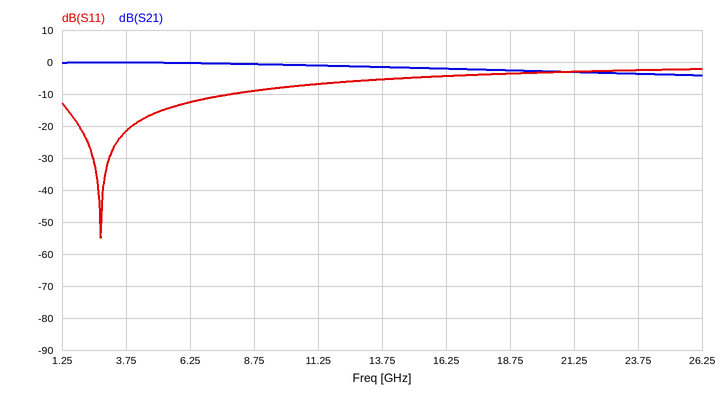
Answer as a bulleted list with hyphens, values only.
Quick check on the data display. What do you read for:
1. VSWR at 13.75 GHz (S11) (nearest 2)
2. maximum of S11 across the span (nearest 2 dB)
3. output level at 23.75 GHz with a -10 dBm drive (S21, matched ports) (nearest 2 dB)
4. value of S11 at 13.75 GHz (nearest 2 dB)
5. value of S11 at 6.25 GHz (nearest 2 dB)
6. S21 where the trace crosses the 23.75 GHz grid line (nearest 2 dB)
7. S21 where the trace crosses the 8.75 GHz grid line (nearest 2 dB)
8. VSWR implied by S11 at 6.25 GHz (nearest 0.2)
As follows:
- 4
- -2 dB
- -14 dBm
- -6 dB
- -12 dB
- -4 dB
- 0 dB
- 1.6
